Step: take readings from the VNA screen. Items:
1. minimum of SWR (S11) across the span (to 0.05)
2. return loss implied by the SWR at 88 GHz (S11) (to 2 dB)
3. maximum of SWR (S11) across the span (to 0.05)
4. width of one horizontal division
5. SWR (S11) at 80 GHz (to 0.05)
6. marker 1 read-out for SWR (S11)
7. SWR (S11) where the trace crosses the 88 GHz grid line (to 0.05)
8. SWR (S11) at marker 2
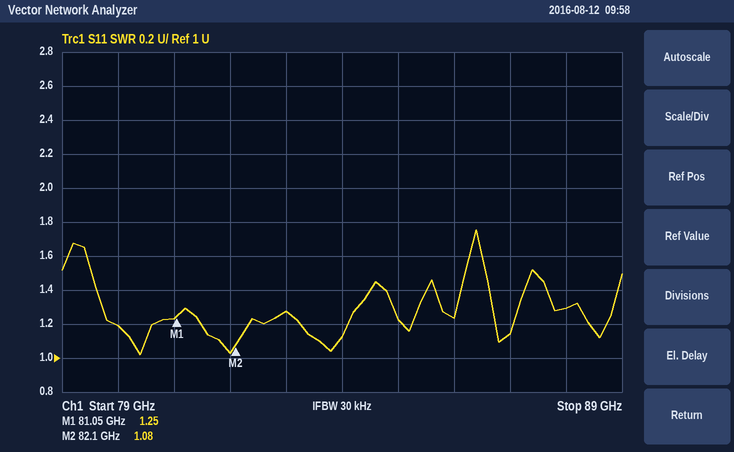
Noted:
1.00
18 dB
1.75
1 GHz
1.20
1.25
1.30
1.08
